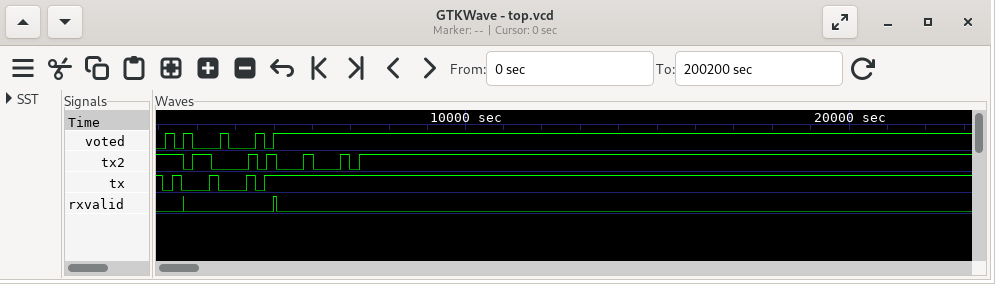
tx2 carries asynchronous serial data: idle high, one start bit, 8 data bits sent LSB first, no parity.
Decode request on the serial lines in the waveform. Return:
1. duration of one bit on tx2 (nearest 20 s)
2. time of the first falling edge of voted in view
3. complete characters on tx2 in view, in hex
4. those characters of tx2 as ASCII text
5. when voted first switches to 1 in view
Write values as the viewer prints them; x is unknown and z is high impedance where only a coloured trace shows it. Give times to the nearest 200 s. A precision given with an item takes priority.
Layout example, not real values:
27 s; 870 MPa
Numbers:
240 s; 2400 s; 43, 44; "CD"; 2200 s
